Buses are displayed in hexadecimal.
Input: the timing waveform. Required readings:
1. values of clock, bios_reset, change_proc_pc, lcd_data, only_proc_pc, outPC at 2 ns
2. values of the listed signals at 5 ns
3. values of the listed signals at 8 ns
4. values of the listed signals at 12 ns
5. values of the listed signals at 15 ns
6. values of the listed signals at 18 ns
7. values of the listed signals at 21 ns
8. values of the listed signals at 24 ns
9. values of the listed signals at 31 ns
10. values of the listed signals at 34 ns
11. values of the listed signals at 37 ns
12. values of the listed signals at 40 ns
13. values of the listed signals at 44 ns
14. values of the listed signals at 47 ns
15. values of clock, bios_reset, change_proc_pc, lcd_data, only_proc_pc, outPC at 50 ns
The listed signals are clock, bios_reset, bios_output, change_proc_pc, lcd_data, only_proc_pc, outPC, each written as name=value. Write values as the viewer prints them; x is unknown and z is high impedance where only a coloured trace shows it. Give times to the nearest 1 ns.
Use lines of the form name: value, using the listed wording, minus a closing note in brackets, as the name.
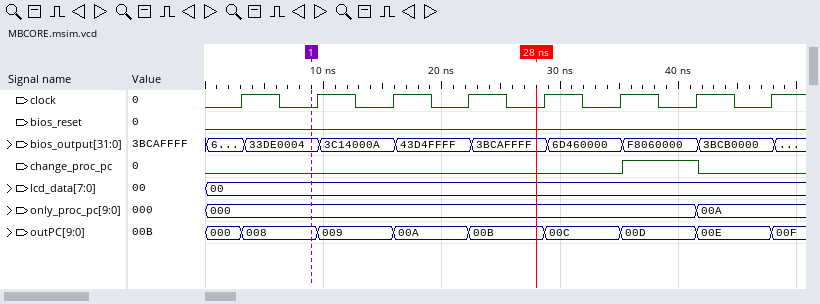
values of clock, bios_reset, change_proc_pc, lcd_data, only_proc_pc, outPC at 2 ns: clock=0, bios_reset=0, change_proc_pc=0, lcd_data=00, only_proc_pc=000, outPC=000
values of the listed signals at 5 ns: clock=1, bios_reset=0, bios_output=33DE0004, change_proc_pc=0, lcd_data=00, only_proc_pc=000, outPC=008
values of the listed signals at 8 ns: clock=0, bios_reset=0, bios_output=33DE0004, change_proc_pc=0, lcd_data=00, only_proc_pc=000, outPC=008
values of the listed signals at 12 ns: clock=1, bios_reset=0, bios_output=3C14000A, change_proc_pc=0, lcd_data=00, only_proc_pc=000, outPC=009
values of the listed signals at 15 ns: clock=0, bios_reset=0, bios_output=3C14000A, change_proc_pc=0, lcd_data=00, only_proc_pc=000, outPC=009
values of the listed signals at 18 ns: clock=1, bios_reset=0, bios_output=43D4FFFF, change_proc_pc=0, lcd_data=00, only_proc_pc=000, outPC=00A
values of the listed signals at 21 ns: clock=0, bios_reset=0, bios_output=43D4FFFF, change_proc_pc=0, lcd_data=00, only_proc_pc=000, outPC=00A
values of the listed signals at 24 ns: clock=1, bios_reset=0, bios_output=3BCAFFFF, change_proc_pc=0, lcd_data=00, only_proc_pc=000, outPC=00B
values of the listed signals at 31 ns: clock=1, bios_reset=0, bios_output=6D460000, change_proc_pc=0, lcd_data=00, only_proc_pc=000, outPC=00C
values of the listed signals at 34 ns: clock=0, bios_reset=0, bios_output=6D460000, change_proc_pc=0, lcd_data=00, only_proc_pc=000, outPC=00C
values of the listed signals at 37 ns: clock=1, bios_reset=0, bios_output=F8060000, change_proc_pc=1, lcd_data=00, only_proc_pc=000, outPC=00D
values of the listed signals at 40 ns: clock=0, bios_reset=0, bios_output=F8060000, change_proc_pc=1, lcd_data=00, only_proc_pc=000, outPC=00D
values of the listed signals at 44 ns: clock=1, bios_reset=0, bios_output=3BCB0000, change_proc_pc=0, lcd_data=00, only_proc_pc=00A, outPC=00E
values of the listed signals at 47 ns: clock=0, bios_reset=0, bios_output=3BCB0000, change_proc_pc=0, lcd_data=00, only_proc_pc=00A, outPC=00E
values of clock, bios_reset, change_proc_pc, lcd_data, only_proc_pc, outPC at 50 ns: clock=1, bios_reset=0, change_proc_pc=0, lcd_data=00, only_proc_pc=00A, outPC=00F
